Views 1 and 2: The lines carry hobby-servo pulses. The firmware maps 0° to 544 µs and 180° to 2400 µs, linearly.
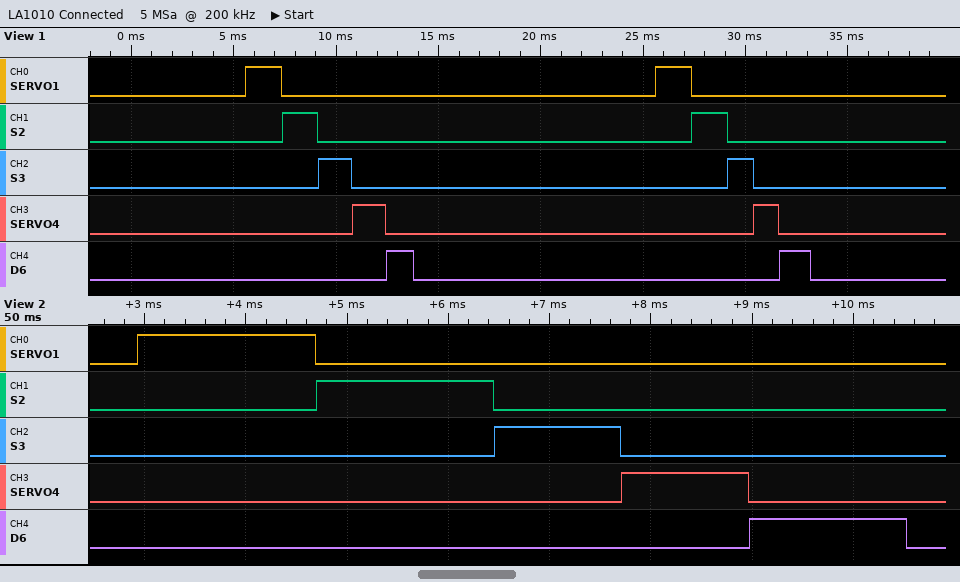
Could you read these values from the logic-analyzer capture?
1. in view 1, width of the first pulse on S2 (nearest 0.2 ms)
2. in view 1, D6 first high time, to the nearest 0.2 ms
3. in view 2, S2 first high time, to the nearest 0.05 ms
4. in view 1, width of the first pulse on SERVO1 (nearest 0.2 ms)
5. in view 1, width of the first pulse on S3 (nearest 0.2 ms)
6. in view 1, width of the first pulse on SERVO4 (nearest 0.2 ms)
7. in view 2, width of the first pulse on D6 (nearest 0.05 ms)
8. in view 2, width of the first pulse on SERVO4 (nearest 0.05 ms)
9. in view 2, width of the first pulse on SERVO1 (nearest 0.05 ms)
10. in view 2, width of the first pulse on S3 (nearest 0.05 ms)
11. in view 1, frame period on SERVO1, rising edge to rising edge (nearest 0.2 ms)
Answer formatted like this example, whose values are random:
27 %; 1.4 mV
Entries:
1.8 ms; 1.4 ms; 1.75 ms; 1.8 ms; 1.6 ms; 1.6 ms; 1.55 ms; 1.25 ms; 1.75 ms; 1.25 ms; 20.0 ms
